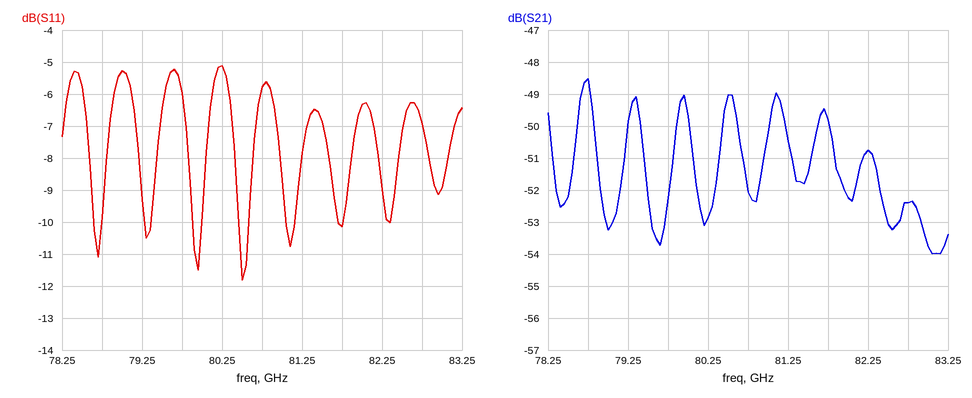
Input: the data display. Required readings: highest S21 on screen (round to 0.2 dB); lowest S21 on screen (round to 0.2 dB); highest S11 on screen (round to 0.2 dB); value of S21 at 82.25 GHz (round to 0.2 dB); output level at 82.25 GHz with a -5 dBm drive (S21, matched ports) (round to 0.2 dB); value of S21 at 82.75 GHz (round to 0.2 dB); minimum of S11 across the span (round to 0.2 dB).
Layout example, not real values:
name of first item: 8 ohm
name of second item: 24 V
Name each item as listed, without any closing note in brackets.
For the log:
highest S21 on screen: -48.6 dB
lowest S21 on screen: -54.0 dB
highest S11 on screen: -5.2 dB
value of S21 at 82.25 GHz: -50.8 dB
output level at 82.25 GHz with a -5 dBm drive (S21, matched ports): -55.8 dBm
value of S21 at 82.75 GHz: -52.4 dB
minimum of S11 across the span: -11.8 dB
